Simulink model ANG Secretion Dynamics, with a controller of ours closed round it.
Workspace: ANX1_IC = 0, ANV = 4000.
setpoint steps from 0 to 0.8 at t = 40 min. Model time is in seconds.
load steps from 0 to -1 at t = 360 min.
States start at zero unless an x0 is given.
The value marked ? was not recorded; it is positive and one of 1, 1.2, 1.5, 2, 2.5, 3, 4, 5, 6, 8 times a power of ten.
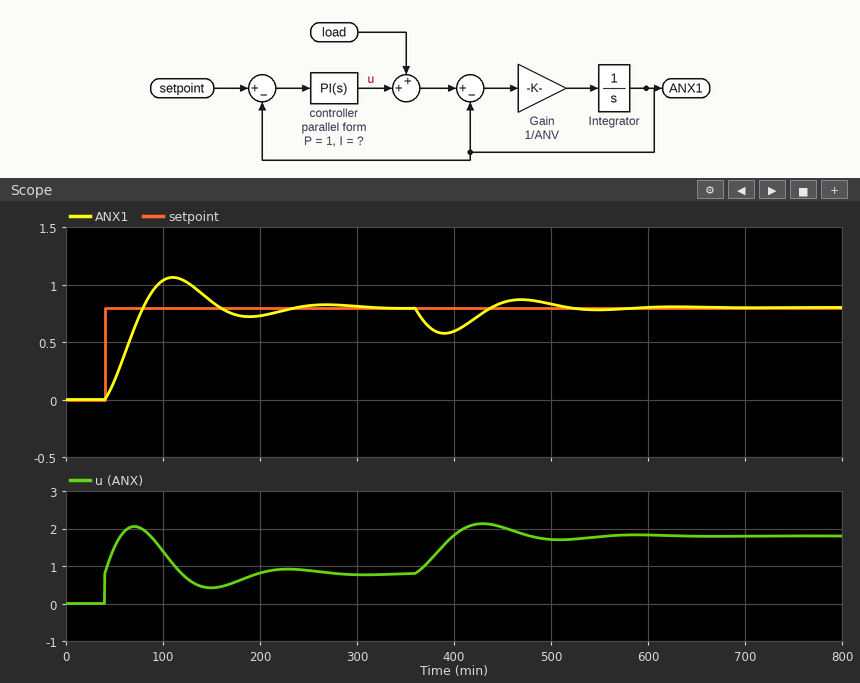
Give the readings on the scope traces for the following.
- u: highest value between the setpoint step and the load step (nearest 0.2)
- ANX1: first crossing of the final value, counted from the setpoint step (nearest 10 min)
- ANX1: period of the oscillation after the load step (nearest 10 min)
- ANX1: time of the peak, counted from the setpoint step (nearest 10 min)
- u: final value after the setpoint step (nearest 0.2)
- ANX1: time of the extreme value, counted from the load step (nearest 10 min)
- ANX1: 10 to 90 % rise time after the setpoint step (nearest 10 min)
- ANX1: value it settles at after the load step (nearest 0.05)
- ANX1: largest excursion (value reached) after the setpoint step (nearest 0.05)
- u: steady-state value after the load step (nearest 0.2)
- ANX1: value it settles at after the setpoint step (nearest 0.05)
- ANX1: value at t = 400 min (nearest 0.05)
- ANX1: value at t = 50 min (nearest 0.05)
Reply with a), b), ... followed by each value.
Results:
a) 2.0
b) 40 min
c) 160 min
d) 70 min
e) 0.8
f) 30 min
g) 30 min
h) 0.80
i) 1.05
j) 1.8
k) 0.80
l) 0.60
m) 0.15
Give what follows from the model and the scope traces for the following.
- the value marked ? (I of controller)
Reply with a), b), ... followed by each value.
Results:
a) 0.002
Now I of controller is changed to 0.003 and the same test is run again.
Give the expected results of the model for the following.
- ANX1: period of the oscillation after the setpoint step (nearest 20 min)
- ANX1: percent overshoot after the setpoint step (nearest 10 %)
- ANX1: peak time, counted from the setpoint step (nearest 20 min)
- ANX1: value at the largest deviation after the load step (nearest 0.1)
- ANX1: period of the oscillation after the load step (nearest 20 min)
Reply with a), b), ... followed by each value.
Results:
a) 120 min
b) 40 %
c) 60 min
d) 0.6
e) 120 min
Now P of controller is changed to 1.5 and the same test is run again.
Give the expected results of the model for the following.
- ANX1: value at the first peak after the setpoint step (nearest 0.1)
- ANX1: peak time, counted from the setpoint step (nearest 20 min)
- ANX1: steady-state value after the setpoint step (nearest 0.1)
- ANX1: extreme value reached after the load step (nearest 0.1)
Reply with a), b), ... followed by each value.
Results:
a) 1.0
b) 60 min
c) 0.8
d) 0.6
